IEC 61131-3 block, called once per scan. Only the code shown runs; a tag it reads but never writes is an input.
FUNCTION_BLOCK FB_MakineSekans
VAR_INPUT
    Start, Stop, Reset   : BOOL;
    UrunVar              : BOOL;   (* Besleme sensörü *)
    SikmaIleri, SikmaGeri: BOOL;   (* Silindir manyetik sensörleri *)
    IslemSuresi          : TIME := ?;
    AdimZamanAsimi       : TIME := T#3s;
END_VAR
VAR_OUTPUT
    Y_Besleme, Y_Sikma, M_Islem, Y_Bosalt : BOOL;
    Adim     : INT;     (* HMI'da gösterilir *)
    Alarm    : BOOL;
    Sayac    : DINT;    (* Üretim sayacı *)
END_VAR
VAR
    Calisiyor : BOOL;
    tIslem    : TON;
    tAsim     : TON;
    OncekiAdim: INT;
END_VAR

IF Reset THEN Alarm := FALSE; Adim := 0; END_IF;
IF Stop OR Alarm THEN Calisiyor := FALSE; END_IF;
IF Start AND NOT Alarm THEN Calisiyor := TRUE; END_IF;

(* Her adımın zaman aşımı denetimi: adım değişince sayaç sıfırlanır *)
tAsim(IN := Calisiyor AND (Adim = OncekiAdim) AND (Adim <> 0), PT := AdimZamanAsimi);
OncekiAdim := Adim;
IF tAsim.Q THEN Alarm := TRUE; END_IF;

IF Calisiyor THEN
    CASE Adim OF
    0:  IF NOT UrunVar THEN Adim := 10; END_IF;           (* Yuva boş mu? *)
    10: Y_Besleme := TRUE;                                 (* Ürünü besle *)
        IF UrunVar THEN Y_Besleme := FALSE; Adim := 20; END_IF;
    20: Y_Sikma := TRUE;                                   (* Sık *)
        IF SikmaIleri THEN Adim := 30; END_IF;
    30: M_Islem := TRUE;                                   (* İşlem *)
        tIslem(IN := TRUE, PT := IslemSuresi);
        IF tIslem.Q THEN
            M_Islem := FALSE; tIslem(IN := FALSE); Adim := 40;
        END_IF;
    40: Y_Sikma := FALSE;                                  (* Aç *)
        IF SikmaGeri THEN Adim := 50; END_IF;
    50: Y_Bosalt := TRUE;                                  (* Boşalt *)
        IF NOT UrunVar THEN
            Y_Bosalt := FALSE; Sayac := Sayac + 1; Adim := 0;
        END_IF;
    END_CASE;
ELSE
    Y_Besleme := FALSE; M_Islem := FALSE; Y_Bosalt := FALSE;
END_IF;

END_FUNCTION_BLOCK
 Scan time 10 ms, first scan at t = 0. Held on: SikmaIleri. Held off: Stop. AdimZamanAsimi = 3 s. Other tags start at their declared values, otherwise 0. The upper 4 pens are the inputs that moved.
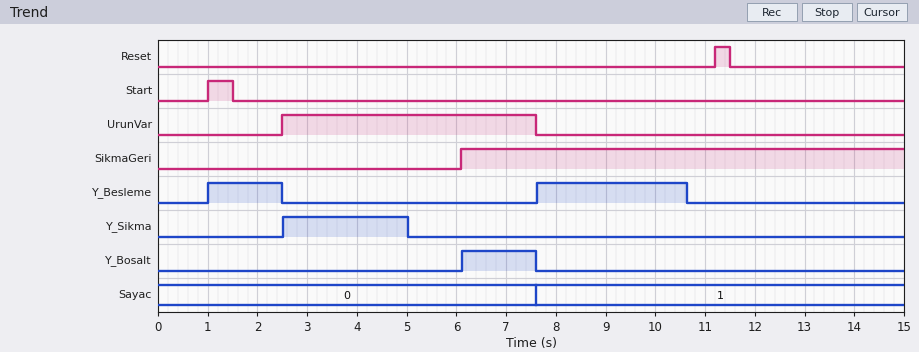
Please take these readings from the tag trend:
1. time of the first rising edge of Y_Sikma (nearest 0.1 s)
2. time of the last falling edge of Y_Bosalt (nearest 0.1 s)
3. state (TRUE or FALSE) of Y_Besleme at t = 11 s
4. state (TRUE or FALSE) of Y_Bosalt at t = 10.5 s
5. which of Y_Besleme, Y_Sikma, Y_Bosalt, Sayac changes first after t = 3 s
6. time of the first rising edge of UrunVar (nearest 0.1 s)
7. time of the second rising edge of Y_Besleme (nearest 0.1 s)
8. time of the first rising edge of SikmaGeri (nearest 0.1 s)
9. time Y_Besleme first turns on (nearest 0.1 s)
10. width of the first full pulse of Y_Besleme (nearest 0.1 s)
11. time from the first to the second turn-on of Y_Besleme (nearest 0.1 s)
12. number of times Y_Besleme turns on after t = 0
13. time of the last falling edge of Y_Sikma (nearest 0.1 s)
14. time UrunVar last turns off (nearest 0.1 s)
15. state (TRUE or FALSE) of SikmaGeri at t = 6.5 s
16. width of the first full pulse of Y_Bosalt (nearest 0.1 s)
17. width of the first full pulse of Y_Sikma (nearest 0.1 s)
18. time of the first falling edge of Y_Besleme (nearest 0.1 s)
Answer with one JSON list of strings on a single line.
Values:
["2.5 s", "7.6 s", "FALSE", "FALSE", "Y_Sikma", "2.5 s", "7.6 s", "6.1 s", "1.0 s", "1.5 s", "6.6 s", "2", "5.0 s", "7.6 s", "TRUE", "1.5 s", "2.5 s", "2.5 s"]
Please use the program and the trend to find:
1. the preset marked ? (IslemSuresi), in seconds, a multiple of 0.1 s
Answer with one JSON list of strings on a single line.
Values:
["2.5 s"]
